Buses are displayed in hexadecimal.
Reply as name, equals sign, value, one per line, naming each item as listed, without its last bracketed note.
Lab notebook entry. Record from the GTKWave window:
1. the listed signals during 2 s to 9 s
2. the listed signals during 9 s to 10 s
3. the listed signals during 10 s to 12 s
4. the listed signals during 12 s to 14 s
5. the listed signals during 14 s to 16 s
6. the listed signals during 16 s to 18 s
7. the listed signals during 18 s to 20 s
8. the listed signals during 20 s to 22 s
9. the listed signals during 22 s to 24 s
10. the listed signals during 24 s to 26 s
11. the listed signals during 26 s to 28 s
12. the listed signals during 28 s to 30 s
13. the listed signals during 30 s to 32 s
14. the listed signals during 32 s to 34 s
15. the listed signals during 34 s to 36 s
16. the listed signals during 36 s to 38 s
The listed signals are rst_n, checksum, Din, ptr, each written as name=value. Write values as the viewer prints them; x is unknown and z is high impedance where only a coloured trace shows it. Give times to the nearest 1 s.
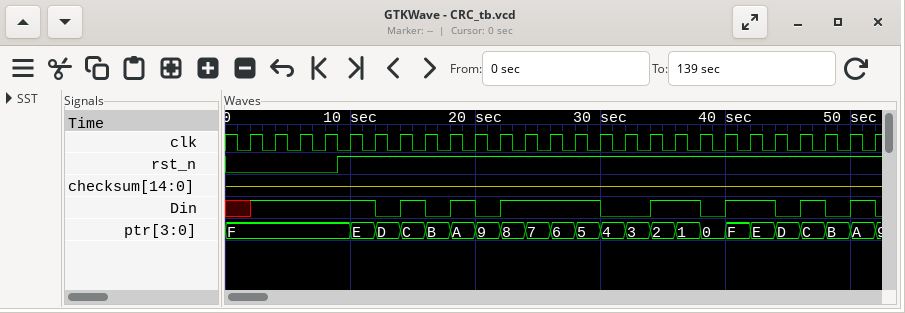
the listed signals during 2 s to 9 s = rst_n=0, checksum=z, Din=1, ptr=F
the listed signals during 9 s to 10 s = rst_n=1, checksum=z, Din=1, ptr=F
the listed signals during 10 s to 12 s = rst_n=1, checksum=z, Din=1, ptr=E
the listed signals during 12 s to 14 s = rst_n=1, checksum=z, Din=0, ptr=D
the listed signals during 14 s to 16 s = rst_n=1, checksum=z, Din=1, ptr=C
the listed signals during 16 s to 18 s = rst_n=1, checksum=z, Din=0, ptr=B
the listed signals during 18 s to 20 s = rst_n=1, checksum=z, Din=1, ptr=A
the listed signals during 20 s to 22 s = rst_n=1, checksum=z, Din=0, ptr=9
the listed signals during 22 s to 24 s = rst_n=1, checksum=z, Din=1, ptr=8
the listed signals during 24 s to 26 s = rst_n=1, checksum=z, Din=1, ptr=7
the listed signals during 26 s to 28 s = rst_n=1, checksum=z, Din=1, ptr=6
the listed signals during 28 s to 30 s = rst_n=1, checksum=z, Din=1, ptr=5
the listed signals during 30 s to 32 s = rst_n=1, checksum=z, Din=0, ptr=4
the listed signals during 32 s to 34 s = rst_n=1, checksum=z, Din=0, ptr=3
the listed signals during 34 s to 36 s = rst_n=1, checksum=z, Din=1, ptr=2
the listed signals during 36 s to 38 s = rst_n=1, checksum=z, Din=1, ptr=1
